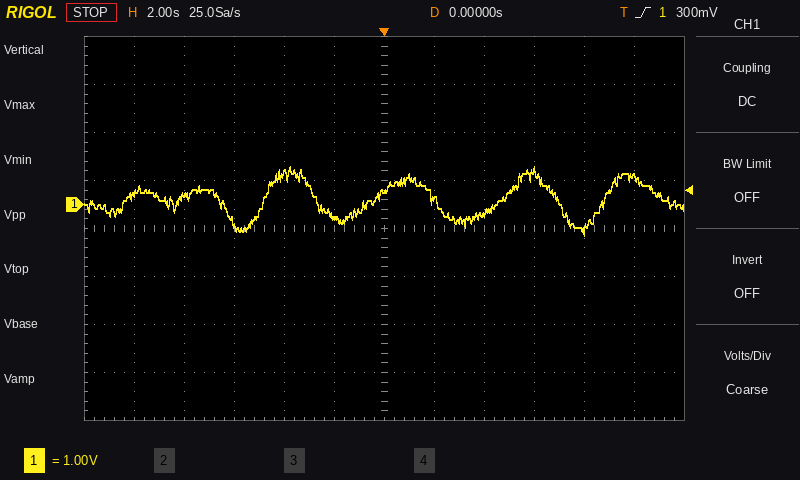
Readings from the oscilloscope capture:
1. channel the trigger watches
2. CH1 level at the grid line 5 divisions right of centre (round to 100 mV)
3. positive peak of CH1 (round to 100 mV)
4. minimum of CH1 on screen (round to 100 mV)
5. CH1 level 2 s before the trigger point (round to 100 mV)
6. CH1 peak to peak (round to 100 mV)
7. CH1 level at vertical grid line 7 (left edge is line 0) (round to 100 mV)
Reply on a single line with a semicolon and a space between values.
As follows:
CH1; 600 mV; 800 mV; -600 mV; -200 mV; 1.4 V; 100 mV
